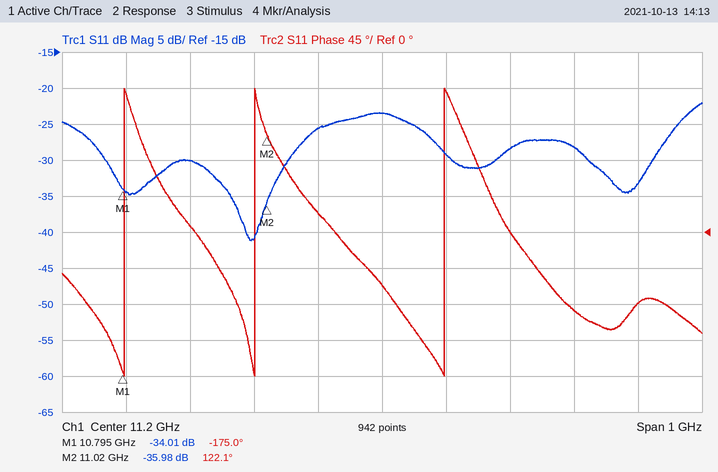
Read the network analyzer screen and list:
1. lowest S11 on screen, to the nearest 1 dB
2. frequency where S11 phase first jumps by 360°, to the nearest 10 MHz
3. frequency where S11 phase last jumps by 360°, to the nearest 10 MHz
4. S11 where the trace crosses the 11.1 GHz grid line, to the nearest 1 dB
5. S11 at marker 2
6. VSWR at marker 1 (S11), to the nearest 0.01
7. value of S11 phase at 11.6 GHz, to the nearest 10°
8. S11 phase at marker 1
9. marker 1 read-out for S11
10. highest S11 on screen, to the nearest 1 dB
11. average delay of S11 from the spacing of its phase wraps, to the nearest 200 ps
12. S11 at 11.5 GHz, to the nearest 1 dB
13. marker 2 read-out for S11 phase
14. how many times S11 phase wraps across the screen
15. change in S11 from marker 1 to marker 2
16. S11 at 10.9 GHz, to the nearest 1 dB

-41 dB
10.80 GHz
11.30 GHz
-26 dB
-35.98 dB
1.04
-90°
-175.0°
-34.01 dB
-22 dB
4.0 ns
-28 dB
122.1°
3
-1.97 dB
-30 dB
